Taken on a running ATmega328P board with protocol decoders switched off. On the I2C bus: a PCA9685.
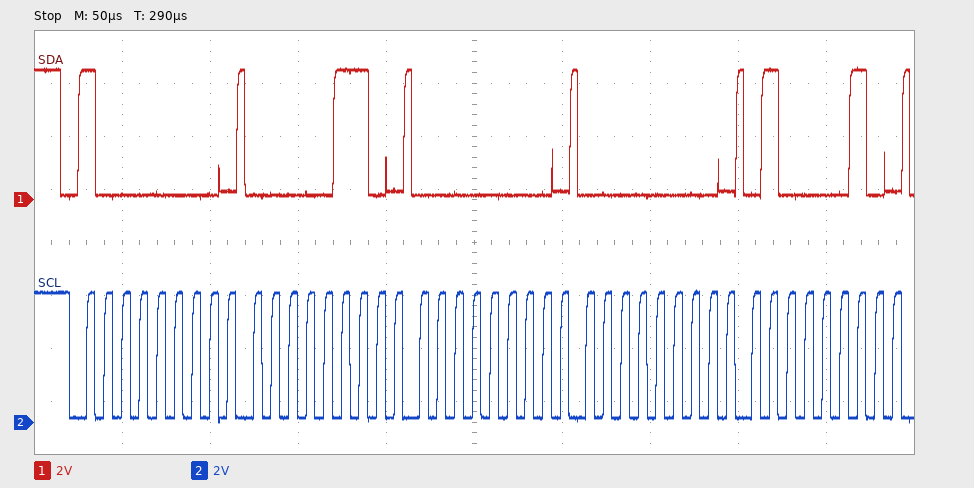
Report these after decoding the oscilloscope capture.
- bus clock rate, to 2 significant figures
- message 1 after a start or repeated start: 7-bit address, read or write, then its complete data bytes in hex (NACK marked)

100 kHz
0x40 write: 06 00 00 42
